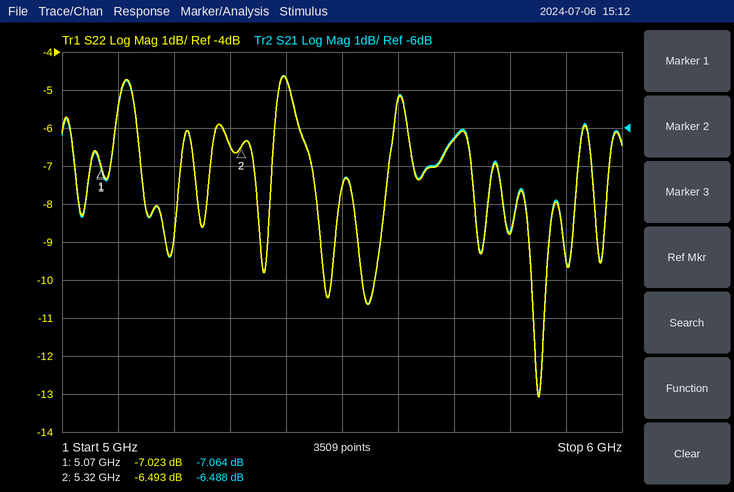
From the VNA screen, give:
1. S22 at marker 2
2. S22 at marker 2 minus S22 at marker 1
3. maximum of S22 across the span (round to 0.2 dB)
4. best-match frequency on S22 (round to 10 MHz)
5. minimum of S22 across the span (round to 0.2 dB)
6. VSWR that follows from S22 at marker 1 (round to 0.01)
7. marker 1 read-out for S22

-6.493 dB
0.530 dB
-4.6 dB
5.85 GHz
-13.0 dB
2.61
-7.023 dB
